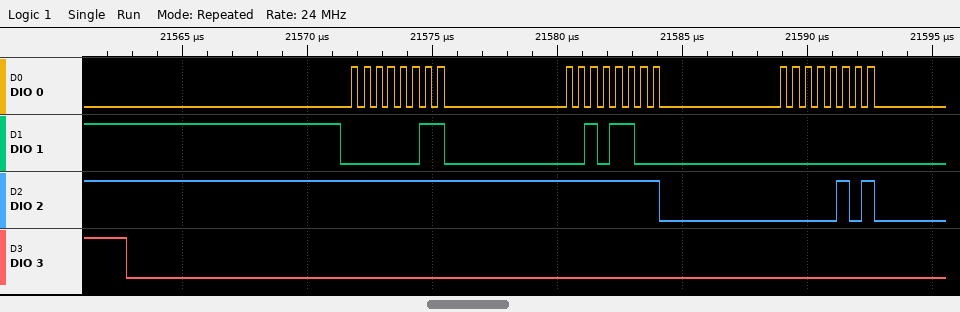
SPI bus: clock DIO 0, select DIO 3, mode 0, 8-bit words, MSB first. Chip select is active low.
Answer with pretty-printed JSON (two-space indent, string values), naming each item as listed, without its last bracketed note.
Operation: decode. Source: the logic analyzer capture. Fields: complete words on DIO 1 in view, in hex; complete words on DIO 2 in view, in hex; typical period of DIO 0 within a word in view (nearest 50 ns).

{
  "complete words on DIO 1 in view, in hex": "03, 2C, 00",
  "complete words on DIO 2 in view, in hex": "FF, FF, 05",
  "typical period of DIO 0 within a word in view": "500 ns"
}
